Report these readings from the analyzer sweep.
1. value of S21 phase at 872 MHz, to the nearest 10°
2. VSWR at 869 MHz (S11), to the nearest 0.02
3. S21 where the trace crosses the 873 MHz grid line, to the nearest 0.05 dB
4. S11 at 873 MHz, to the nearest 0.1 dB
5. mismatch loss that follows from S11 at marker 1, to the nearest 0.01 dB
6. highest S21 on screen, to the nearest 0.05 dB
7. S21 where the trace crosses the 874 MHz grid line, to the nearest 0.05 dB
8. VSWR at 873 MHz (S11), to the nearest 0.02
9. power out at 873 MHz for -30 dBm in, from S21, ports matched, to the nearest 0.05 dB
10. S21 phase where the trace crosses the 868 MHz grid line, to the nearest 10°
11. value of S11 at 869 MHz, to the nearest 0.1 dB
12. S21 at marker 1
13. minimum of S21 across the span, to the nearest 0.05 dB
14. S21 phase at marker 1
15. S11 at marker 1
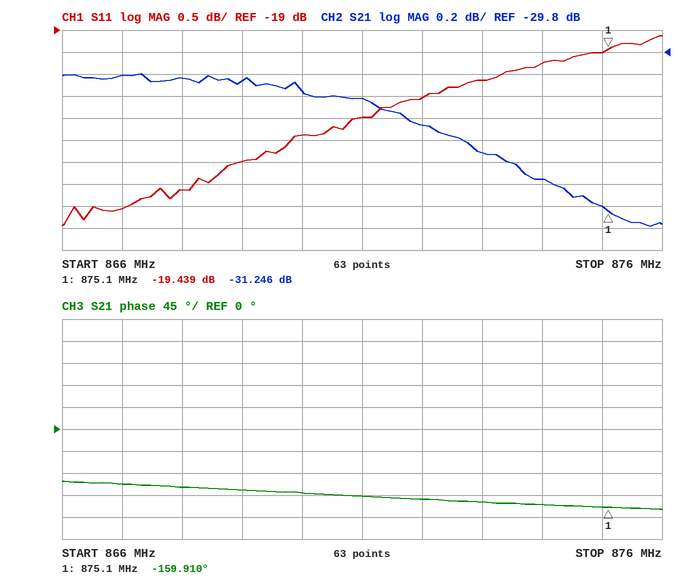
-140°
1.18
-30.70 dB
-20.1 dB
0.05 dB
-30.00 dB
-30.95 dB
1.22
-60.70 dBm
-120°
-22.0 dB
-31.246 dB
-31.40 dB
-159.910°
-19.439 dB
